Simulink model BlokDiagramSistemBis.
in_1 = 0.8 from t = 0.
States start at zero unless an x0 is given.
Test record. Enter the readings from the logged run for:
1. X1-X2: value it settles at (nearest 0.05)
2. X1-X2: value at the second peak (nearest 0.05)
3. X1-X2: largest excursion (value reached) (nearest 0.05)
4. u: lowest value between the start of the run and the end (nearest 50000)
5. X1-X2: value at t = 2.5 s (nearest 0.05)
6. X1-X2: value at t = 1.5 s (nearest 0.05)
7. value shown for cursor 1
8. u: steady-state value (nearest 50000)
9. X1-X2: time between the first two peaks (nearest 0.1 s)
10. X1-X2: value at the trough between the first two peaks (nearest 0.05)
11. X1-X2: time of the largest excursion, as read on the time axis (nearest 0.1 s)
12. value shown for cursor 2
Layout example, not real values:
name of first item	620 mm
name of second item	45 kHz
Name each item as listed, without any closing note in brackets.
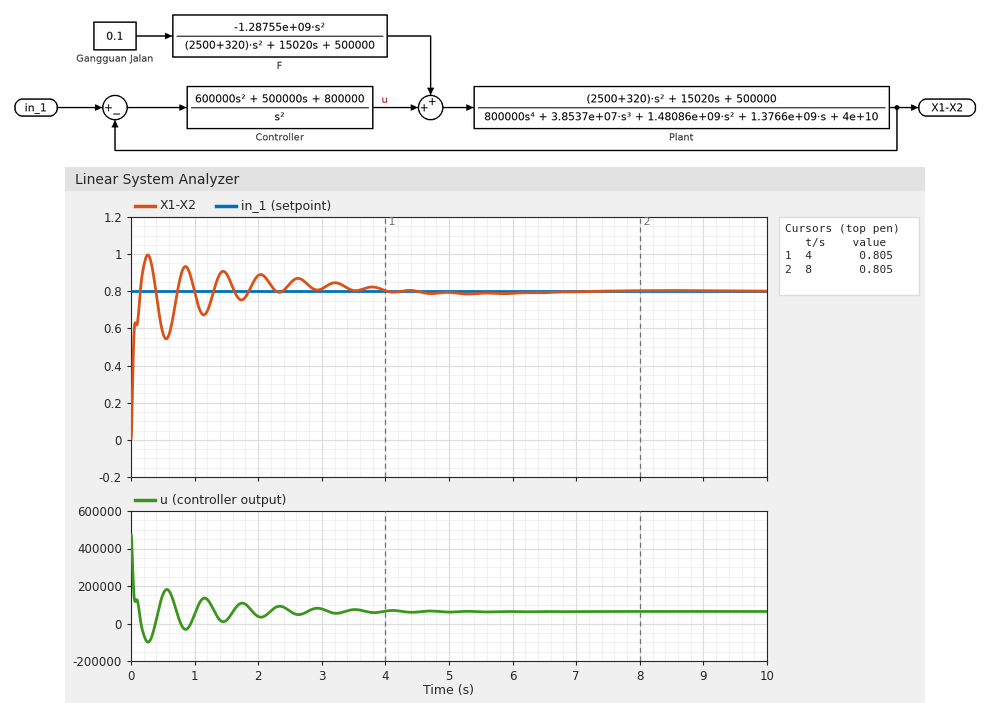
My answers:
X1-X2: value it settles at	0.80
X1-X2: value at the second peak	0.95
X1-X2: largest excursion (value reached)	1.00
u: lowest value between the start of the run and the end	-100000
X1-X2: value at t = 2.5 s	0.85
X1-X2: value at t = 1.5 s	0.90
value shown for cursor 1	0.805
u: steady-state value	50000
X1-X2: time between the first two peaks	0.6 s
X1-X2: value at the trough between the first two peaks	0.55
X1-X2: time of the largest excursion, as read on the time axis	0.3 s
value shown for cursor 2	0.805
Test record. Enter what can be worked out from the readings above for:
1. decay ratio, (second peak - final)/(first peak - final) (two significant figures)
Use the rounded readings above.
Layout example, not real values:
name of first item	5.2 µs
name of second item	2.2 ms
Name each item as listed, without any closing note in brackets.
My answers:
decay ratio, (second peak - final)/(first peak - final)	0.75
